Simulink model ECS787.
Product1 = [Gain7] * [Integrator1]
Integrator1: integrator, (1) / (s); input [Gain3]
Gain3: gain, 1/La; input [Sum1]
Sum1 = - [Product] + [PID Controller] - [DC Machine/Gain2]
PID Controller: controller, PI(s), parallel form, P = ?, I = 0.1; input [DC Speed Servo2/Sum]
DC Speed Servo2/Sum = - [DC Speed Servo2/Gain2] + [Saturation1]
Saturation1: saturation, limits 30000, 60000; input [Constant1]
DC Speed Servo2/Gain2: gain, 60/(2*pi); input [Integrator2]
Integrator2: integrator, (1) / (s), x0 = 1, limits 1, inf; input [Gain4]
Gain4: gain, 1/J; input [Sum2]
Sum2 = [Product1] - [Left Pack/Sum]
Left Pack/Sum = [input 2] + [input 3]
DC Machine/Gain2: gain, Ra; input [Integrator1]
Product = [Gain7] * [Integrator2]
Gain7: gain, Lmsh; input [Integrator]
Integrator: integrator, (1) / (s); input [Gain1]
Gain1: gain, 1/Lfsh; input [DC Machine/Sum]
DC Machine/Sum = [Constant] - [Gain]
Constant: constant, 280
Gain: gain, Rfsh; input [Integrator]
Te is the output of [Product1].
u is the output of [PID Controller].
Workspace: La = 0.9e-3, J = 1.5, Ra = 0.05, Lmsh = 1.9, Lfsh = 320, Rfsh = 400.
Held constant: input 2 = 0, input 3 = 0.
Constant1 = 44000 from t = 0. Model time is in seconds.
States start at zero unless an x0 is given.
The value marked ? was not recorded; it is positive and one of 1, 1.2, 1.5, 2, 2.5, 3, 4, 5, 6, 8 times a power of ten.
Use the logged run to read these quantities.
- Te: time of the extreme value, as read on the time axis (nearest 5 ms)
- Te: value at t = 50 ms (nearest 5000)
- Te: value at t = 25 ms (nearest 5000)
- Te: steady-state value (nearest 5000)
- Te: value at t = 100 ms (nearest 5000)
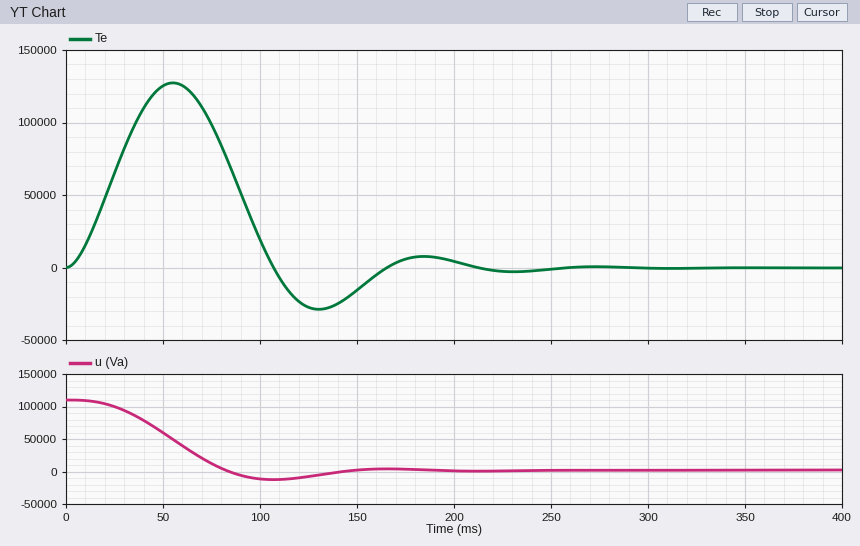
55 ms
125000
65000
0
20000
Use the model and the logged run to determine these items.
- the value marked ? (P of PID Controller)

2.5
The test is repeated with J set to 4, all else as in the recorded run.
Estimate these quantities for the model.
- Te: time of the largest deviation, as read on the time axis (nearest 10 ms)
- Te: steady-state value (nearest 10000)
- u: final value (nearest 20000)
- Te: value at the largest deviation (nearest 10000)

80 ms
0
0
190000
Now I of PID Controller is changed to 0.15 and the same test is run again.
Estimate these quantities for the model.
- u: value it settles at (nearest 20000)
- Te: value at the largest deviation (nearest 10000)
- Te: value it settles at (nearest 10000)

0
130000
0
